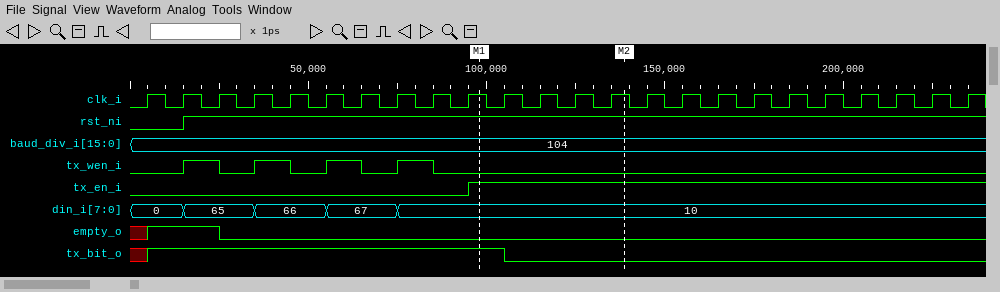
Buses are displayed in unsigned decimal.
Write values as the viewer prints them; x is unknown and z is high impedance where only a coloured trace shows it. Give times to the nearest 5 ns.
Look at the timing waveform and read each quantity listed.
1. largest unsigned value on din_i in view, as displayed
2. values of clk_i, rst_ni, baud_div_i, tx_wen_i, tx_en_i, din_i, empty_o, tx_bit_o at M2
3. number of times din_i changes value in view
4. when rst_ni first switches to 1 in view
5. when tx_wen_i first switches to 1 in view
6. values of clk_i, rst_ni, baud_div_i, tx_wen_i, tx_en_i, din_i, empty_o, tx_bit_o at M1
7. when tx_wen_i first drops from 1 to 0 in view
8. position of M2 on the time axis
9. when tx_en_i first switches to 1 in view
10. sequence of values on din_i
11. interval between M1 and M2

67
clk_i=1, rst_ni=1, baud_div_i=104, tx_wen_i=0, tx_en_i=1, din_i=10, empty_o=0, tx_bit_o=0
4
15 ns
15 ns
clk_i=1, rst_ni=1, baud_div_i=104, tx_wen_i=0, tx_en_i=1, din_i=10, empty_o=0, tx_bit_o=1
25 ns
140 ns
95 ns
0, 65, 66, 67, 10
40 ns
